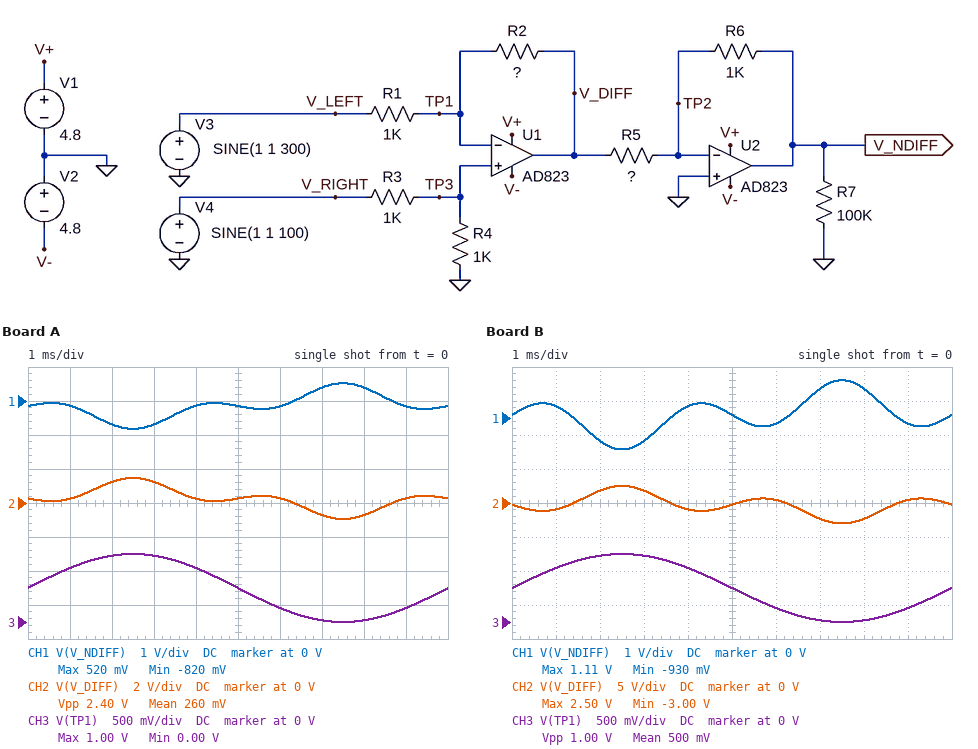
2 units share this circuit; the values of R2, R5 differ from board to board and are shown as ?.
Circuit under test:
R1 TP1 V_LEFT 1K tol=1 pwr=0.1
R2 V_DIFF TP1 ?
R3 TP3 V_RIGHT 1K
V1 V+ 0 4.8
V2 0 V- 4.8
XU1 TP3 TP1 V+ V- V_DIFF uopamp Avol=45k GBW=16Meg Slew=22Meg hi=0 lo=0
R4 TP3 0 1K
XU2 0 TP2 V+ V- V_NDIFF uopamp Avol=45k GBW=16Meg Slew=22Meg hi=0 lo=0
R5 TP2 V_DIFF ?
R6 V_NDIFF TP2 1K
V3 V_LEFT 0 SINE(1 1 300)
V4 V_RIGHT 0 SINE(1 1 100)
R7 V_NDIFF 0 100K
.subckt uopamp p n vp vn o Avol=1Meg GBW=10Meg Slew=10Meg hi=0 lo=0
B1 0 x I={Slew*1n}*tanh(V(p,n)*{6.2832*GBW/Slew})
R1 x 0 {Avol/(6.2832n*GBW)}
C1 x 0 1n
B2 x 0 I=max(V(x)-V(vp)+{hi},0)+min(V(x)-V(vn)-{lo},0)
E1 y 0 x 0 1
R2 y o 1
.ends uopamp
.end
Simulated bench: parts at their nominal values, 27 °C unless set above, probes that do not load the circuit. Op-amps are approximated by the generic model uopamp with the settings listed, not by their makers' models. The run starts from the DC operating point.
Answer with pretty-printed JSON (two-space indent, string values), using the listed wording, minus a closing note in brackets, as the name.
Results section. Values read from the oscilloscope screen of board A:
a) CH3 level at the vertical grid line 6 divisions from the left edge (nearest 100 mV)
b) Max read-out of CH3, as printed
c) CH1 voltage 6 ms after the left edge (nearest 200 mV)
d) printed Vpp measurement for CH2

{
  "CH3 level at the vertical grid line 6 divisions from the left edge": "200 mV",
  "Max read-out of CH3, as printed": "1.00 V",
  "CH1 voltage 6 ms after the left edge": "-200 mV",
  "printed Vpp measurement for CH2": "2.40 V"
}
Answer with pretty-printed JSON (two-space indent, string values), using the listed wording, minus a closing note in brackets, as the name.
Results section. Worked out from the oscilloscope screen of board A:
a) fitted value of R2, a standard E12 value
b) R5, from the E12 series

{
  "fitted value of R2, a standard E12 value": "470 Ω",
  "R5, from the E12 series": "1.8 kΩ"
}
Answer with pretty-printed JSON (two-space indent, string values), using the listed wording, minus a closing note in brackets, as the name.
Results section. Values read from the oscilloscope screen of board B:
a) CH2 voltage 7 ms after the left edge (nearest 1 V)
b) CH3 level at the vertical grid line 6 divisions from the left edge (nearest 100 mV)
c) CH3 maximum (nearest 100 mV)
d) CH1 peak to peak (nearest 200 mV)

{
  "CH2 voltage 7 ms after the left edge": "-2 V",
  "CH3 level at the vertical grid line 6 divisions from the left edge": "200 mV",
  "CH3 maximum": "1.0 V",
  "CH1 peak to peak": "2.0 V"
}
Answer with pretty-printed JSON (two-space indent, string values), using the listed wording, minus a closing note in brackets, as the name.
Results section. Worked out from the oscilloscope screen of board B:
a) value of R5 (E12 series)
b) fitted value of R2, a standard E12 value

{
  "value of R5": "2.7 kΩ",
  "fitted value of R2, a standard E12 value": "1.5 kΩ"
}
